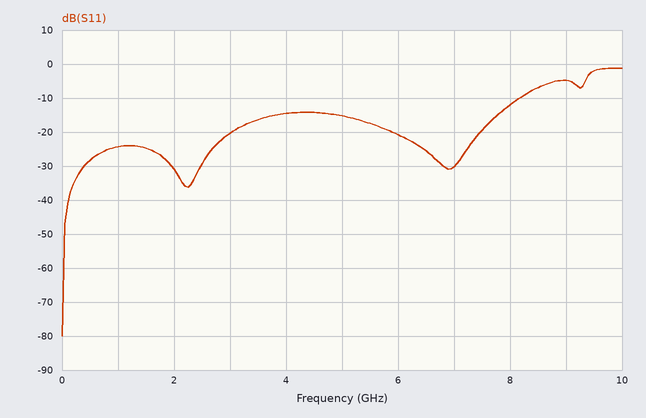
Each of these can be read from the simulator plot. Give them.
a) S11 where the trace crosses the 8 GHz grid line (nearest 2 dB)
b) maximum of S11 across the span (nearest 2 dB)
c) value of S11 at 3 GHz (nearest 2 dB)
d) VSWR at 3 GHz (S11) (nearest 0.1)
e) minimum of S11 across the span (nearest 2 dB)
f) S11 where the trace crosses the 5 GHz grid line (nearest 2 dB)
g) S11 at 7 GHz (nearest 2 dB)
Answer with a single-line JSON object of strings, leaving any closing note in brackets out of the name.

{"S11 where the trace crosses the 8 GHz grid line": "-12 dB", "maximum of S11 across the span": "-2 dB", "value of S11 at 3 GHz": "-20 dB", "VSWR at 3 GHz (S11)": "1.2", "minimum of S11 across the span": "-80 dB", "S11 where the trace crosses the 5 GHz grid line": "-16 dB", "S11 at 7 GHz": "-30 dB"}
